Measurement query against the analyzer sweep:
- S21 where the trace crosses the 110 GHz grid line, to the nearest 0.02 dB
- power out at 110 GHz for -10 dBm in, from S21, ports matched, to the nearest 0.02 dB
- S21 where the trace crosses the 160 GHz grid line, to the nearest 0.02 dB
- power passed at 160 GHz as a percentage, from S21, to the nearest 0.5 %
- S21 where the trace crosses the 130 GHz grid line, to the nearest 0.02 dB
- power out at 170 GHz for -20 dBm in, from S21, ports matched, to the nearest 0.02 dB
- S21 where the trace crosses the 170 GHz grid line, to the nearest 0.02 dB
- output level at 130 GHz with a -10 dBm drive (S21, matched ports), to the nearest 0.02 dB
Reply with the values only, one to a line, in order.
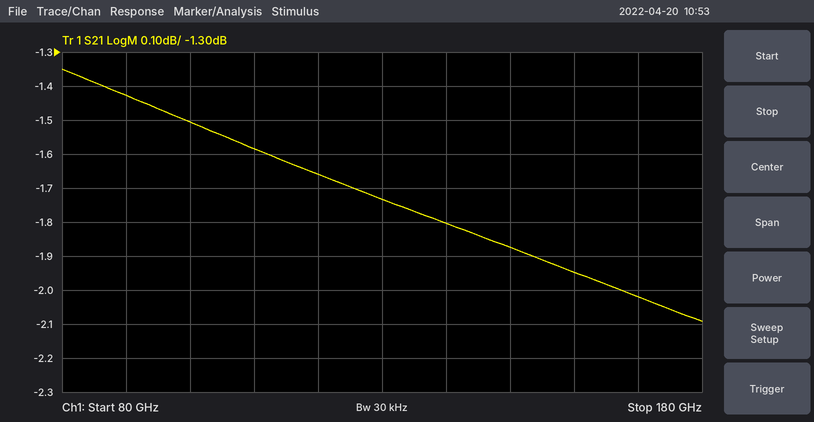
-1.58 dB
-11.58 dBm
-1.94 dB
64.0 %
-1.74 dB
-22.02 dBm
-2.02 dB
-11.74 dBm
